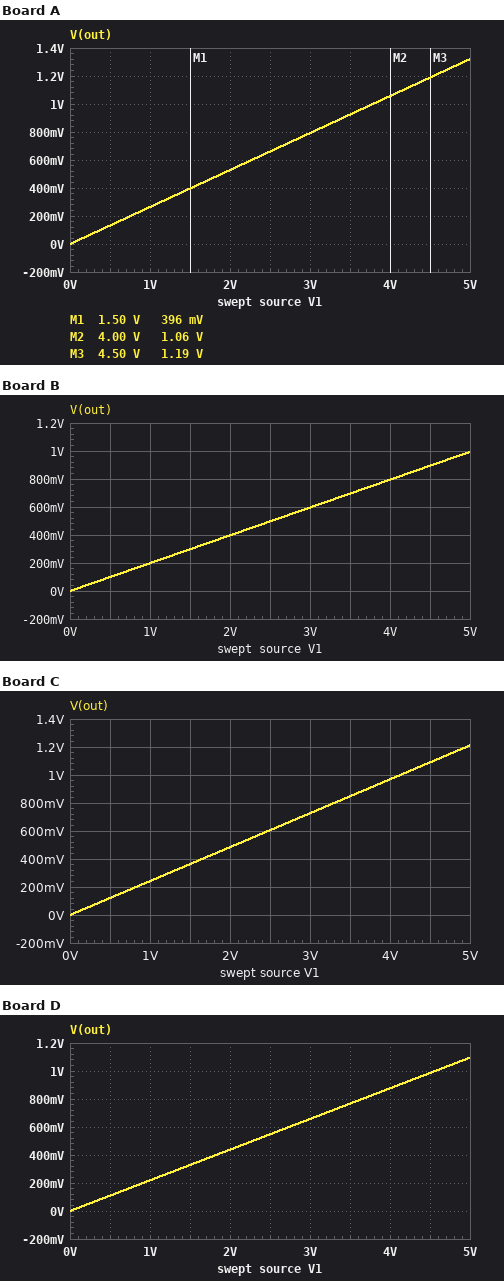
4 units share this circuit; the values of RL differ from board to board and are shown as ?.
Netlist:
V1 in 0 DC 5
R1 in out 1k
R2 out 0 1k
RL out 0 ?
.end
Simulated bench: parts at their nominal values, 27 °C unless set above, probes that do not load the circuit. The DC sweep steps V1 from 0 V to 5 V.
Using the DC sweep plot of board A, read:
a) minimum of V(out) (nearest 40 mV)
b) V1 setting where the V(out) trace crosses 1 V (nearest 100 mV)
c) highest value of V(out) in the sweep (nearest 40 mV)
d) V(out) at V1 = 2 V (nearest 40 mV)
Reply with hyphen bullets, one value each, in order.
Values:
- 0 V
- 3.8 V
- 1.32 V
- 520 mV
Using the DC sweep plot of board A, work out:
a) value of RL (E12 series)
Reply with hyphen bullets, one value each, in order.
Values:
- 560 Ω
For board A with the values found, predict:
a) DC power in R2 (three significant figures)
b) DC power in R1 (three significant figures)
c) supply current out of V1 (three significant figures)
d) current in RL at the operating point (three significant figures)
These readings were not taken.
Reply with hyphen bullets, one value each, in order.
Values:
- 1.74 mW
- 13.5 mW
- 3.68 mA
- 2.36 mA
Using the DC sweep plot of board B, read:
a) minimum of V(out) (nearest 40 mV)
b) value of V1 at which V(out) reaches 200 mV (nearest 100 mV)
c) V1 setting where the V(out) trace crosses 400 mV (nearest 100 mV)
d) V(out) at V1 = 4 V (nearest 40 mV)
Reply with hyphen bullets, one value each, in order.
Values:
- 0 V
- 1.0 V
- 2.0 V
- 800 mV
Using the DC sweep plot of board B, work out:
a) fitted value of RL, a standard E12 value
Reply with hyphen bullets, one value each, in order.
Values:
- 330 Ω
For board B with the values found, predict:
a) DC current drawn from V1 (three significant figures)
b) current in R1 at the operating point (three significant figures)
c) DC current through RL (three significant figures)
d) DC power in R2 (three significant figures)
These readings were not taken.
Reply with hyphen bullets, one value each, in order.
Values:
- 4.01 mA
- 4.01 mA
- 3.01 mA
- 988 µW
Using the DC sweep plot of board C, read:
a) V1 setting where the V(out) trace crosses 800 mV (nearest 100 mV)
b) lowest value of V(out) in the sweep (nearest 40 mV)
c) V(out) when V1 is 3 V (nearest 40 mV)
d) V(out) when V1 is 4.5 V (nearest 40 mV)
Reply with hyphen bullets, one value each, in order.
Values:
- 3.3 V
- 0 V
- 720 mV
- 1.08 V
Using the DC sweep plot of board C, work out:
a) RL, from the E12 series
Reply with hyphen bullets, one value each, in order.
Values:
- 470 Ω
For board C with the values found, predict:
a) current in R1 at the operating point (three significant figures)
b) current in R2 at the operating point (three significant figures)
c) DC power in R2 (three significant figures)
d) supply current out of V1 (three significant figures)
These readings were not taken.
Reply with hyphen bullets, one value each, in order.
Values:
- 3.79 mA
- 1.21 mA
- 1.47 mW
- 3.79 mA
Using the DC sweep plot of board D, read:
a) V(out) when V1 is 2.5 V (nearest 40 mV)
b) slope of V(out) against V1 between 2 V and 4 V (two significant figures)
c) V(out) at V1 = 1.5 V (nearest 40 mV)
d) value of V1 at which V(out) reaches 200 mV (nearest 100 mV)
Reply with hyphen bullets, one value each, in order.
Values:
- 560 mV
- 0.22 V/V
- 320 mV
- 900 mV
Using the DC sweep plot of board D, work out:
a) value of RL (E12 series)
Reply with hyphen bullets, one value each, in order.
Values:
- 390 Ω
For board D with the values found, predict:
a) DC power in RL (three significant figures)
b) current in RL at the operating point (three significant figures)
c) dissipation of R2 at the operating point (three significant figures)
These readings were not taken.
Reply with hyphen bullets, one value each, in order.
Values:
- 3.08 mW
- 2.81 mA
- 1.20 mW
